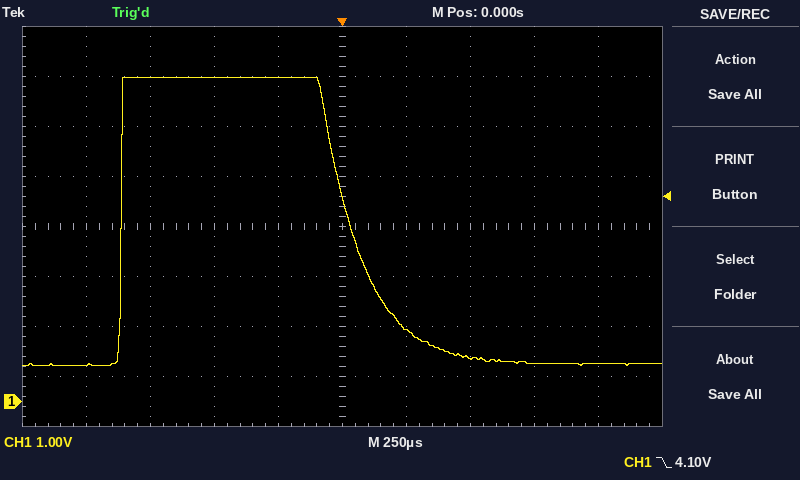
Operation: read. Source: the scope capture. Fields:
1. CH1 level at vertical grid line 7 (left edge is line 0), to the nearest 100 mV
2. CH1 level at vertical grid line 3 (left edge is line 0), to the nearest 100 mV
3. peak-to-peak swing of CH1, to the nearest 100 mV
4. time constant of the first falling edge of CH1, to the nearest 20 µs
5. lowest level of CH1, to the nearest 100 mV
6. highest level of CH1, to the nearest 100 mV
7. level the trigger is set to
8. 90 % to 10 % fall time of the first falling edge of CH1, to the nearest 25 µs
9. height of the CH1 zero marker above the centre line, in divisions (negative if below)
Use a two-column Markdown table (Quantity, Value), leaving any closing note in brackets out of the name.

| Quantity | Value |
|---|---|
| CH1 level at vertical grid line 7 (left edge is line 0), to the nearest 100 mV | 900 mV |
| CH1 level at vertical grid line 3 (left edge is line 0), to the nearest 100 mV | 6.5 V |
| peak-to-peak swing of CH1, to the nearest 100 mV | 5.8 V |
| time constant of the first falling edge of CH1, to the nearest 20 µs | 160 µs |
| lowest level of CH1, to the nearest 100 mV | 700 mV |
| highest level of CH1, to the nearest 100 mV | 6.5 V |
| level the trigger is set to | 4.10 V |
| 90 % to 10 % fall time of the first falling edge of CH1, to the nearest 25 µs | 350 µs |
| height of the CH1 zero marker above the centre line, in divisions | -3.5 div |
